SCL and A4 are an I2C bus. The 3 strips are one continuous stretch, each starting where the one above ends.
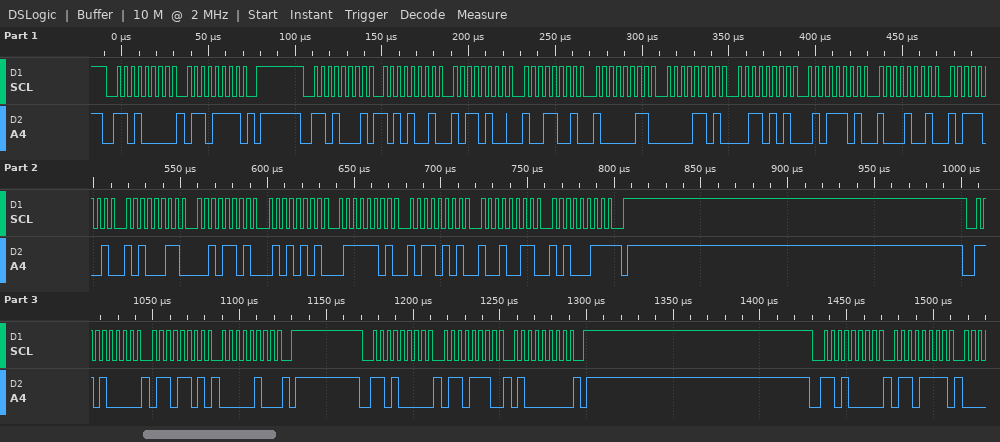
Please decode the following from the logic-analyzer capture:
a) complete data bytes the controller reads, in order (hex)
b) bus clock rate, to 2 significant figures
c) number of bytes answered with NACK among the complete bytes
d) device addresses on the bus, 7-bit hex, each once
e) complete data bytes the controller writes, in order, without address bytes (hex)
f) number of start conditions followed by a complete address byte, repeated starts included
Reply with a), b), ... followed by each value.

a) A9 B4 99 83 0D 35 5D 89 B9 A3 2D 55 7D B5 93 A3
b) 250 kHz
c) 1
d) 0x68
e) 6F 6D 04 6E 40 6F
f) 5
